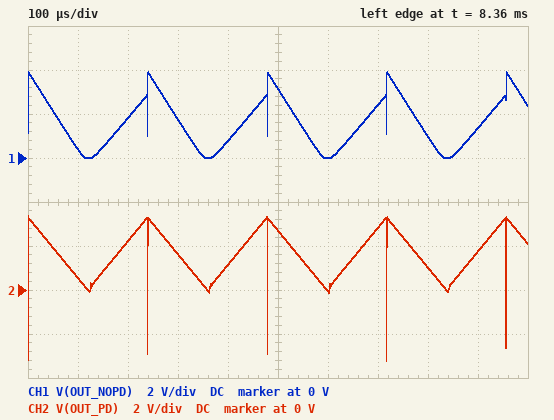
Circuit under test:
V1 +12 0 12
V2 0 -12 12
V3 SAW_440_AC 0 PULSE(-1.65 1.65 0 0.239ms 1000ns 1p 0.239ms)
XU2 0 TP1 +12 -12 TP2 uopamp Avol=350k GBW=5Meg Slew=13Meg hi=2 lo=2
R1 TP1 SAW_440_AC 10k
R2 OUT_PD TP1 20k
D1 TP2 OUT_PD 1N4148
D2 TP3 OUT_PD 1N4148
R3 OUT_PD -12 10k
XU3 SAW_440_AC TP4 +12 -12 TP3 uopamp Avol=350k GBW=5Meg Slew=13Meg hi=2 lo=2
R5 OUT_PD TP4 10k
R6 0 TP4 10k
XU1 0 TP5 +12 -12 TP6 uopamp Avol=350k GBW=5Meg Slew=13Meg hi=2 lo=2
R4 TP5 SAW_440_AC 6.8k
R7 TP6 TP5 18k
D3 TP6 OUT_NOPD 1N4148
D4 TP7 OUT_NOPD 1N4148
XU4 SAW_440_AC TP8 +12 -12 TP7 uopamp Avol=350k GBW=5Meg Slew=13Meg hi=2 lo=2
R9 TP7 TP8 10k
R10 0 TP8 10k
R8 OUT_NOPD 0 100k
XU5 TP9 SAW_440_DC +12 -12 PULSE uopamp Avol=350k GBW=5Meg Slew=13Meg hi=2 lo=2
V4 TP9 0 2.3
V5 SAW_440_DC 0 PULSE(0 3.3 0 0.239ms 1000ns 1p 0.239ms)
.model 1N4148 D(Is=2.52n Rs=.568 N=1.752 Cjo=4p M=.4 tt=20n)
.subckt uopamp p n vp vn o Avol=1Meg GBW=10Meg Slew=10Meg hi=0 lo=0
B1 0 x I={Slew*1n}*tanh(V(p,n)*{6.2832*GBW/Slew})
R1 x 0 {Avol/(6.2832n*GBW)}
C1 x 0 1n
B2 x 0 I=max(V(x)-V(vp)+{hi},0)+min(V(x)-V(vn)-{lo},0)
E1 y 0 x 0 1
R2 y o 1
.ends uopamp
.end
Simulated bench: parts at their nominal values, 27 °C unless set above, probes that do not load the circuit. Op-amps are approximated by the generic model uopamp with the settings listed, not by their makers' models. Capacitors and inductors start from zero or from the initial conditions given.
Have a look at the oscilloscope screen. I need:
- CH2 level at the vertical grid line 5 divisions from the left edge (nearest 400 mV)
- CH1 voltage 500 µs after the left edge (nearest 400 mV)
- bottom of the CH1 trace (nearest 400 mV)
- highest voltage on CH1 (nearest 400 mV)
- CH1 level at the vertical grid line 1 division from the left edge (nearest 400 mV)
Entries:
2.8 V
3.2 V
0 V
4.0 V
400 mV
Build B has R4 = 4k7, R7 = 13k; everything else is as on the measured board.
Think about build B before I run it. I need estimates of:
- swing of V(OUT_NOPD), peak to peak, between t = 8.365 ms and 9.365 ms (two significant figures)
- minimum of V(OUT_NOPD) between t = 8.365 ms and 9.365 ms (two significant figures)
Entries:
4.1 V
-4.1 mV
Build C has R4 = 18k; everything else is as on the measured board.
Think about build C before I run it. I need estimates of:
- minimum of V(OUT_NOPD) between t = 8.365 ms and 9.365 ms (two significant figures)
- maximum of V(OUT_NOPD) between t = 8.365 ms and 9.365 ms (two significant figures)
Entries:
5.2 mV
2.9 V
